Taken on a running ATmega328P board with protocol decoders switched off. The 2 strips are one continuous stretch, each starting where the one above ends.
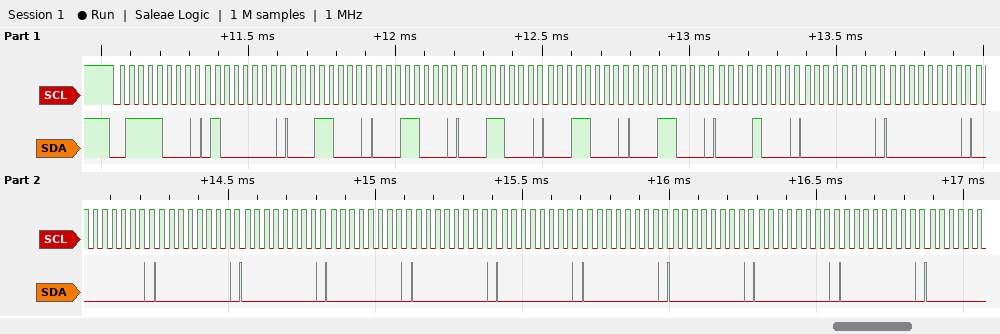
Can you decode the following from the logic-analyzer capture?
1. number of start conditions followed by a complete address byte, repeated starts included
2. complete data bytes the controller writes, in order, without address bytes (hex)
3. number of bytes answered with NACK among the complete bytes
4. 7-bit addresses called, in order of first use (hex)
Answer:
1
40 18 18 18 18 18 08 00 00 00 00 00 00 00 00 00 00 00 00
0
0x3C
